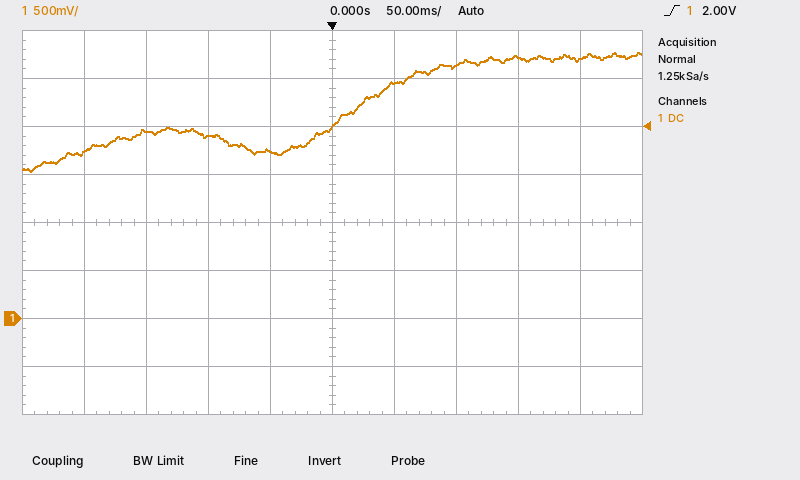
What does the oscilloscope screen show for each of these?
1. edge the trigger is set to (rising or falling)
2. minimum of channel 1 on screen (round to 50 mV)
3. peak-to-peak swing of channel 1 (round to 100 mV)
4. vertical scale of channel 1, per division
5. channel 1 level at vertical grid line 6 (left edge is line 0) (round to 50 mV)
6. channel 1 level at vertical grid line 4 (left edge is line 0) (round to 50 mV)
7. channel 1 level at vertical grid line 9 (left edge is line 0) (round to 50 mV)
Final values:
rising
1.55 V
1.20 V
500 mV
2.45 V
1.75 V
2.70 V
